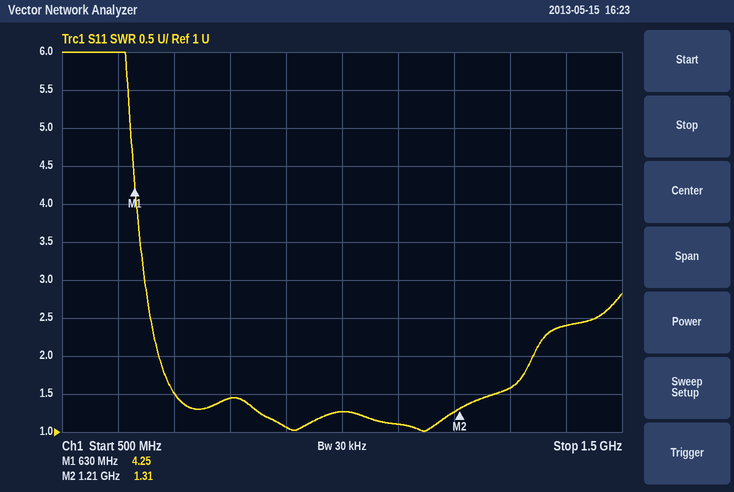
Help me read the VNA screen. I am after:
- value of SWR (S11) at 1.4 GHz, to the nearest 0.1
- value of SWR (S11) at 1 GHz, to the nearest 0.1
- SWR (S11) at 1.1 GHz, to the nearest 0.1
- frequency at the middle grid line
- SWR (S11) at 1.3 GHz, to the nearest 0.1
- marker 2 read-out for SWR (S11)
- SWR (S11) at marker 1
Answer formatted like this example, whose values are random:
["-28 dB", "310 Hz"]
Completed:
["2.4", "1.3", "1.1", "1 GHz", "1.6", "1.31", "4.25"]
